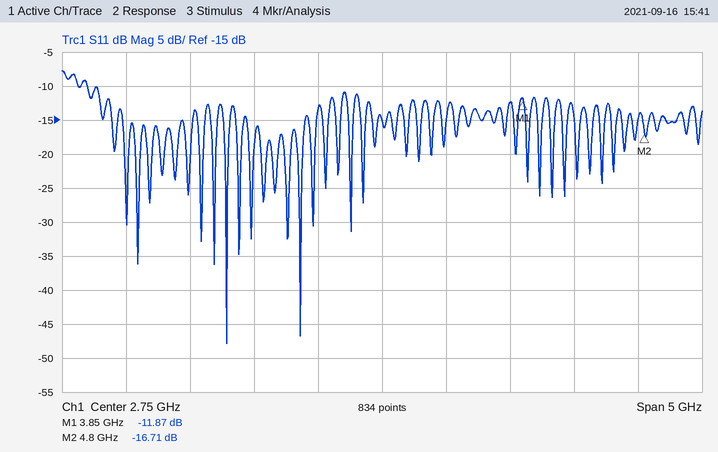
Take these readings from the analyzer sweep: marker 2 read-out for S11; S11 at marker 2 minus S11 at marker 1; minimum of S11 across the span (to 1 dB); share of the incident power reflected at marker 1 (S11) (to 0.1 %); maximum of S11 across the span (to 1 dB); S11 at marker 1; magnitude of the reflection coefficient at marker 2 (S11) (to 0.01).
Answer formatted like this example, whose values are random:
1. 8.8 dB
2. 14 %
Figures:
1. -16.71 dB
2. -4.84 dB
3. -48 dB
4. 6.5 %
5. -8 dB
6. -11.87 dB
7. 0.15
